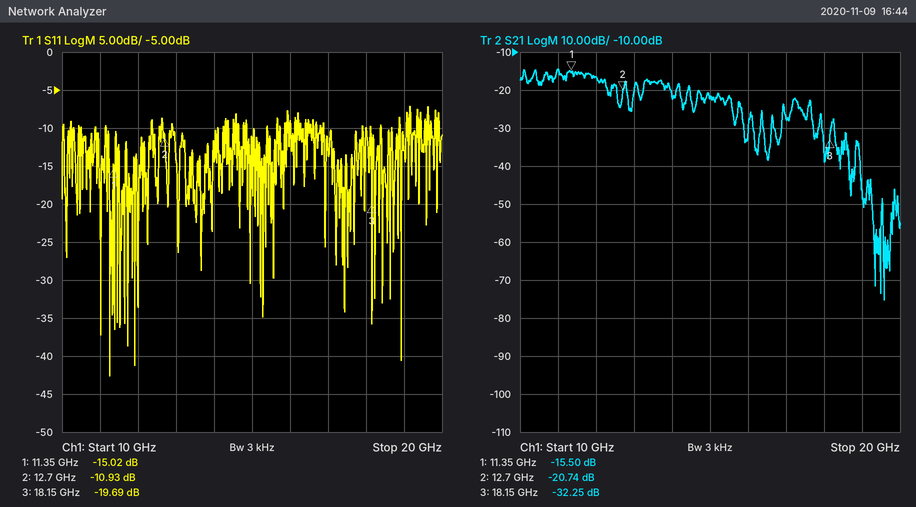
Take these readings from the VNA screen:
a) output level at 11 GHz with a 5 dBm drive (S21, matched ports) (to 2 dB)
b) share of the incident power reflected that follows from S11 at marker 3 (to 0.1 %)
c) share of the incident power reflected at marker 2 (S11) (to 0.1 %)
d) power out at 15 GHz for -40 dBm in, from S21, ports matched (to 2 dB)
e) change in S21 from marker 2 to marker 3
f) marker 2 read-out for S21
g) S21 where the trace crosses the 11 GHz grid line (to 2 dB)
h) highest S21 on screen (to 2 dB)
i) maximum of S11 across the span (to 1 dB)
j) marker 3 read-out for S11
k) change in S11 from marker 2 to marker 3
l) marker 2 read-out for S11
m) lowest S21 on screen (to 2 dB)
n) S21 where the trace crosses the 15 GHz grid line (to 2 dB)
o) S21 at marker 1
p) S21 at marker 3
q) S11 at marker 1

-10 dBm
1.1 %
8.1 %
-62 dBm
-11.51 dB
-20.74 dB
-14 dB
-14 dB
-7 dB
-19.69 dB
-8.76 dB
-10.93 dB
-76 dB
-22 dB
-15.50 dB
-32.25 dB
-15.02 dB
